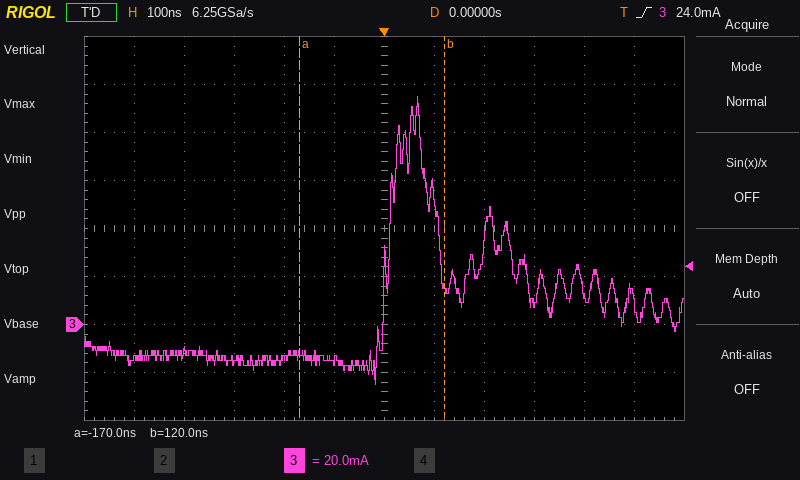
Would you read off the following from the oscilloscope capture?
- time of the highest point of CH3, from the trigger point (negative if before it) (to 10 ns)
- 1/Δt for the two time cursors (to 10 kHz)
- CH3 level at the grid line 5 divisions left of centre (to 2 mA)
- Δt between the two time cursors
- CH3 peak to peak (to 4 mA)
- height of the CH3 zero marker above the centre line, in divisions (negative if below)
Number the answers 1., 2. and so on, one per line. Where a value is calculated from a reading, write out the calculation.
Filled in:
1. +70 ns
2. 1 / 290 ns ≈ 3.45 MHz
3. -14 mA
4. 120 ns − (-170 ns) = 290 ns
5. 120 mA
6. -2.0 div
